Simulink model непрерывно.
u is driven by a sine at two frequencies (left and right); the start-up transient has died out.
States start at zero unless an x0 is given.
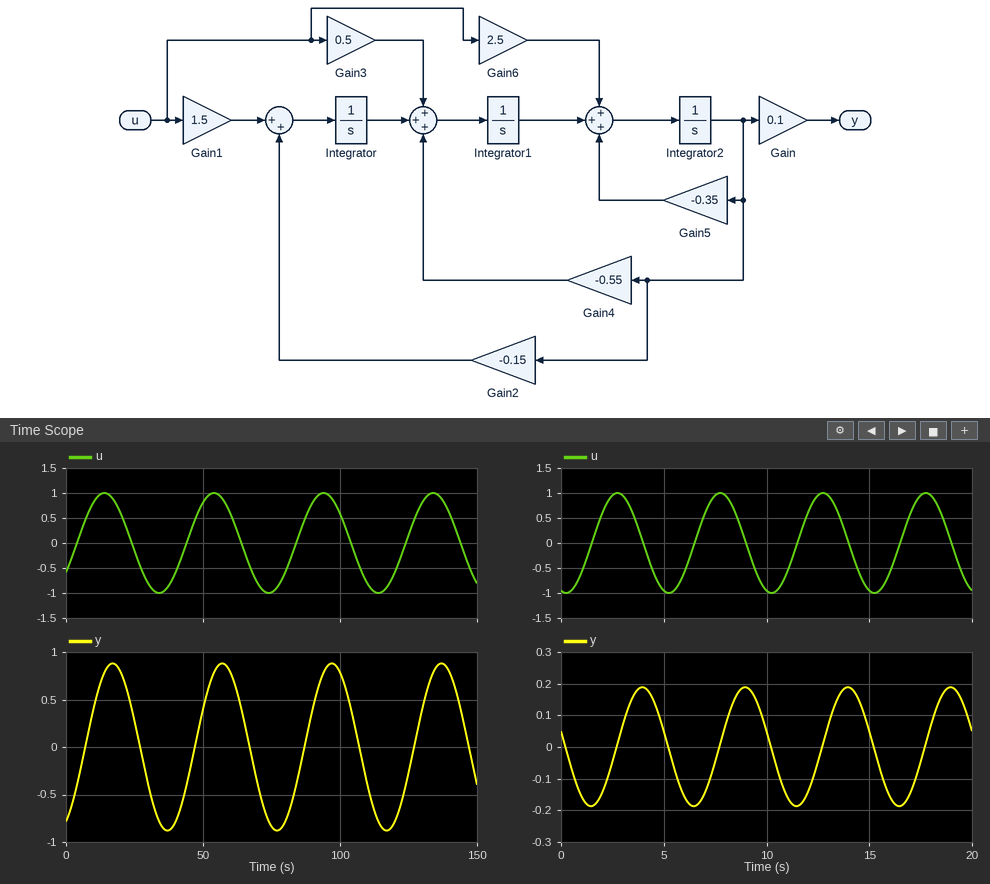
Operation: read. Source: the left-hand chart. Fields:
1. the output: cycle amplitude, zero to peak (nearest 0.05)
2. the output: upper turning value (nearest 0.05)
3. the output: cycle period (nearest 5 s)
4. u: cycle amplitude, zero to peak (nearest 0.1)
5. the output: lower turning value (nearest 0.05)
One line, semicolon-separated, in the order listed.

0.90; 0.90; 40 s; 1.0; -0.90
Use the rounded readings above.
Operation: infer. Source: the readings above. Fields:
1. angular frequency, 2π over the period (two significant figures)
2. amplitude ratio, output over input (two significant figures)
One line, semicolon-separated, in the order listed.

0.16 rad/s; 0.90
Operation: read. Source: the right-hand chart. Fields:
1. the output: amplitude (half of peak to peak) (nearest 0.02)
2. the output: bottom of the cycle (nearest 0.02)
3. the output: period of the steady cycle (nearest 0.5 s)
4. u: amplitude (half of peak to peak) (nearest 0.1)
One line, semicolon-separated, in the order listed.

0.18; -0.18; 5.0 s; 1.0
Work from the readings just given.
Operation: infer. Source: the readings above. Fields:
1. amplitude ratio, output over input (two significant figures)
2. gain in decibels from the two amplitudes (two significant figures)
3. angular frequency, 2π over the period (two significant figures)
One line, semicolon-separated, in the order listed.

0.18; -15 dB; 1.3 rad/s
